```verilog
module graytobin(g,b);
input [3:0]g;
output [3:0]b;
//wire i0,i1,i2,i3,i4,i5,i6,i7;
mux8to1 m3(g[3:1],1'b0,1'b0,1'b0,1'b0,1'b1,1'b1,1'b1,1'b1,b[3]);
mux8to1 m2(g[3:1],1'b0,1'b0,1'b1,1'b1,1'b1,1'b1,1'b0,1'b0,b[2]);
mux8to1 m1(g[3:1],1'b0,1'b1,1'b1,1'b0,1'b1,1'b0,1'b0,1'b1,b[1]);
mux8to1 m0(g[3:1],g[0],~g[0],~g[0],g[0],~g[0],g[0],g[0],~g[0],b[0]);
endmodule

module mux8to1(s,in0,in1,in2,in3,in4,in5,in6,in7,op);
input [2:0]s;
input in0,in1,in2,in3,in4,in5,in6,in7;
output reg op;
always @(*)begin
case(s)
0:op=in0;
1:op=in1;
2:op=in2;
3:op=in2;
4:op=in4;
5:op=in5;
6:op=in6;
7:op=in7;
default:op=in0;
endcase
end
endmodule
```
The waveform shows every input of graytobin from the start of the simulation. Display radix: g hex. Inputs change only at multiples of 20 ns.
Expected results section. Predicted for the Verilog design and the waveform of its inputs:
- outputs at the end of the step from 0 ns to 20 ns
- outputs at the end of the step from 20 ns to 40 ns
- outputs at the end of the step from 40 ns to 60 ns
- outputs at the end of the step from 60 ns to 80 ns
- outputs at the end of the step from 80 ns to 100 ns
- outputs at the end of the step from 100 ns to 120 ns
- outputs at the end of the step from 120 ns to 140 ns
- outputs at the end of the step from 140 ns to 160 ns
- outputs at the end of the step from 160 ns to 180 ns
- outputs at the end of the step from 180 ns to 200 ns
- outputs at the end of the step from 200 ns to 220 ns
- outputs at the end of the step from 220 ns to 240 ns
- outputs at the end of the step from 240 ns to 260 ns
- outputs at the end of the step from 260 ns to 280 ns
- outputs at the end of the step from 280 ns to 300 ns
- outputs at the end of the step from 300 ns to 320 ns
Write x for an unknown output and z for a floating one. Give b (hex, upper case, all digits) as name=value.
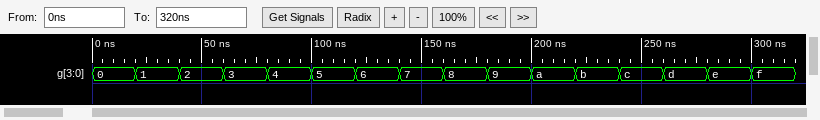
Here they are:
b=0
b=1
b=3
b=2
b=7
b=6
b=7
b=6
b=F
b=E
b=C
b=D
b=8
b=9
b=B
b=A
